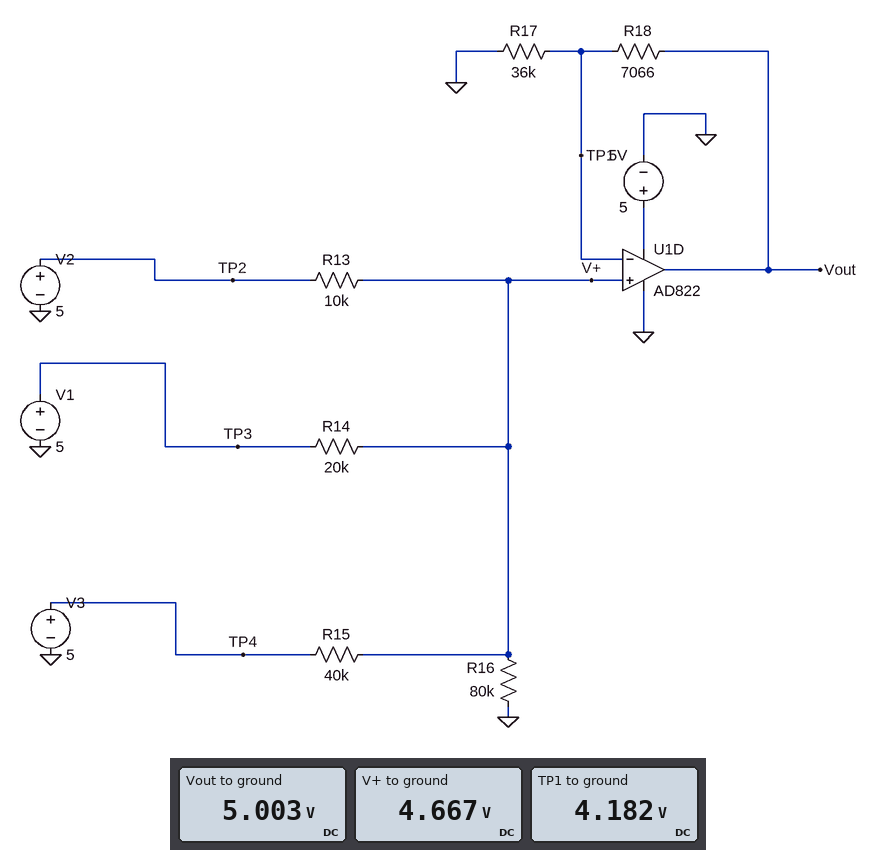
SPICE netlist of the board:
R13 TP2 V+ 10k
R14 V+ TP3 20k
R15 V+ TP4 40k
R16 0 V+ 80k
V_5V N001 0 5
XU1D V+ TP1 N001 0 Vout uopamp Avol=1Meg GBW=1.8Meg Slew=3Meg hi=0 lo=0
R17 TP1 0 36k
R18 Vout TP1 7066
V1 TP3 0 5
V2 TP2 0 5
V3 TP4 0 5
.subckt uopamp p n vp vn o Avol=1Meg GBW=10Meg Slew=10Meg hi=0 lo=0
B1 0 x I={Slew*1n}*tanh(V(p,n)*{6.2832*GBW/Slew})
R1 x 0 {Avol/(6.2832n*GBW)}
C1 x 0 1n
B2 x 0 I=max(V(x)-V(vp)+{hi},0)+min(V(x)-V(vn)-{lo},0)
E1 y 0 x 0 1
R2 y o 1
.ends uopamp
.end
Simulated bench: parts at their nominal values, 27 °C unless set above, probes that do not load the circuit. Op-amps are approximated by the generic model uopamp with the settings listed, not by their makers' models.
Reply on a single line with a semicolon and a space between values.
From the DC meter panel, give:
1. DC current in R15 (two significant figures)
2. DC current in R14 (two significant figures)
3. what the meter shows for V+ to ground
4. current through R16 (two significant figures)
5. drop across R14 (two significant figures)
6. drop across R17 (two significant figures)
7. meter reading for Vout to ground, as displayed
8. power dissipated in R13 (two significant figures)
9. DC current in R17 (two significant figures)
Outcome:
8.3 µA; 17 µA; 4.667 V; 58 µA; 330 mV; 4.2 V; 5.003 V; 11 µW; 120 µA
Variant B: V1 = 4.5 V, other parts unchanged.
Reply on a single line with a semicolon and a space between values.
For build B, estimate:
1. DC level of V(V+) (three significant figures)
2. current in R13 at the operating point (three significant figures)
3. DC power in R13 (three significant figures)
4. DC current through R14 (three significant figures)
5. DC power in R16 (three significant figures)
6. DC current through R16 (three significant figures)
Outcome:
4.53 V; 46.7 µA; 21.8 µW; 1.67 µA; 257 µW; 56.7 µA
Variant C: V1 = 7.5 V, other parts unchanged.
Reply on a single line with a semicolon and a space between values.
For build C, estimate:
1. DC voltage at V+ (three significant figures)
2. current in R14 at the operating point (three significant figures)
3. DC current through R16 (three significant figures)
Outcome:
5.33 V; 108 µA; 66.7 µA
